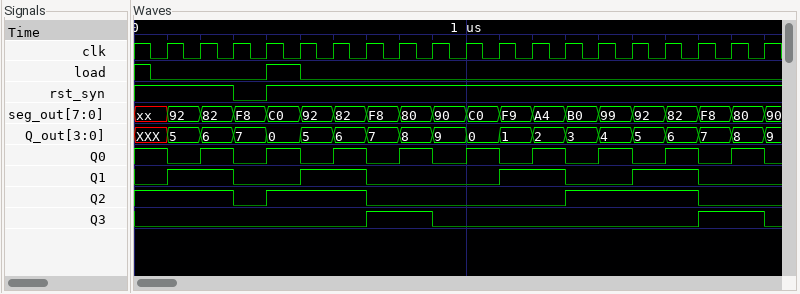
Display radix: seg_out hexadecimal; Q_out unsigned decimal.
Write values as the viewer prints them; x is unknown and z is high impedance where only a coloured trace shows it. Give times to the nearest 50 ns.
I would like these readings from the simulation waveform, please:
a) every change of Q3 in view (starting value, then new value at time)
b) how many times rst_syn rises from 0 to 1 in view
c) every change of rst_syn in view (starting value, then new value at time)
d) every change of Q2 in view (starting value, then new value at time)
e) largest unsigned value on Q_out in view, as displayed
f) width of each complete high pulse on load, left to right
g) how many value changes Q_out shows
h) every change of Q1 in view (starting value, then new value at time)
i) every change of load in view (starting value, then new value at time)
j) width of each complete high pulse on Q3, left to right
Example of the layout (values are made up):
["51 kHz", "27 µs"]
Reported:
["0, 1 at 700 ns, 0 at 900 ns, 1 at 1700 ns, 0 at 1900 ns", "1", "1, 0 at 300 ns, 1 at 400 ns", "1, 0 at 300 ns, 1 at 400 ns, 0 at 700 ns, 1 at 1300 ns, 0 at 1700 ns", "9", "100 ns", "19", "0, 1 at 100 ns, 0 at 300 ns, 1 at 500 ns, 0 at 700 ns, 1 at 1100 ns, 0 at 1300 ns, 1 at 1500 ns, 0 at 1700 ns", "1, 0 at 50 ns, 1 at 400 ns, 0 at 500 ns", "200 ns, 200 ns"]
